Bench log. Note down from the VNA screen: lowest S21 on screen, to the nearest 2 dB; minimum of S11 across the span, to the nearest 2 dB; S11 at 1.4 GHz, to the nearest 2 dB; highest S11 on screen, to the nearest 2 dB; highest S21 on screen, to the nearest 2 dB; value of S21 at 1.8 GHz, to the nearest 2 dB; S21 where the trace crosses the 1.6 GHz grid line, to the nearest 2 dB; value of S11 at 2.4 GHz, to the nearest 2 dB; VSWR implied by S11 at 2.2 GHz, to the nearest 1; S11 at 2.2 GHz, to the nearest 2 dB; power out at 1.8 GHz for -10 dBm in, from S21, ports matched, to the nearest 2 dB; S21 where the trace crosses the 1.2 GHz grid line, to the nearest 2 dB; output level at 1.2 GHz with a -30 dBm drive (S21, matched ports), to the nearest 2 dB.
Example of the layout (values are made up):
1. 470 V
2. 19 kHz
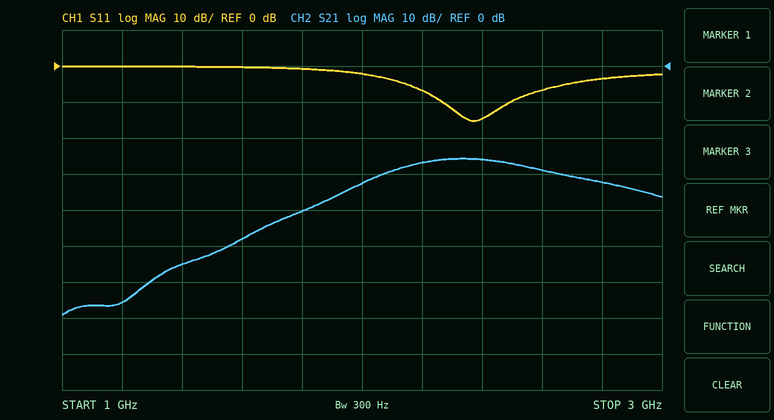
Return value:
1. -70 dB
2. -16 dB
3. 0 dB
4. 0 dB
5. -26 dB
6. -40 dB
7. -48 dB
8. -14 dB
9. 3
10. -6 dB
11. -50 dBm
12. -66 dB
13. -96 dBm
